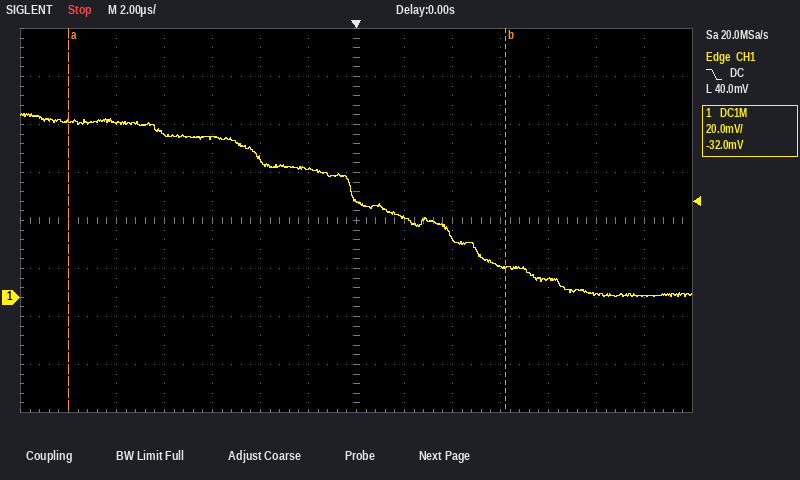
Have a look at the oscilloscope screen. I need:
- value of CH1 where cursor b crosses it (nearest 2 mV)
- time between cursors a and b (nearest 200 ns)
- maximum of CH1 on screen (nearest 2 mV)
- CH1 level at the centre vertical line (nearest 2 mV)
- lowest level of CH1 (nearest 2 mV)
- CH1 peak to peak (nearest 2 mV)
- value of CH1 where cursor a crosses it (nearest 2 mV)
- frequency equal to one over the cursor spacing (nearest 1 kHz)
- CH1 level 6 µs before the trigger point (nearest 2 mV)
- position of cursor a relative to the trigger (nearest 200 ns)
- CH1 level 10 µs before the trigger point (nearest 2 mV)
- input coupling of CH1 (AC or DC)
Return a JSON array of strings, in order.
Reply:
["12 mV", "18.2 µs", "76 mV", "40 mV", "0 mV", "76 mV", "74 mV", "55 kHz", "66 mV", "-12.0 µs", "72 mV", "DC"]
